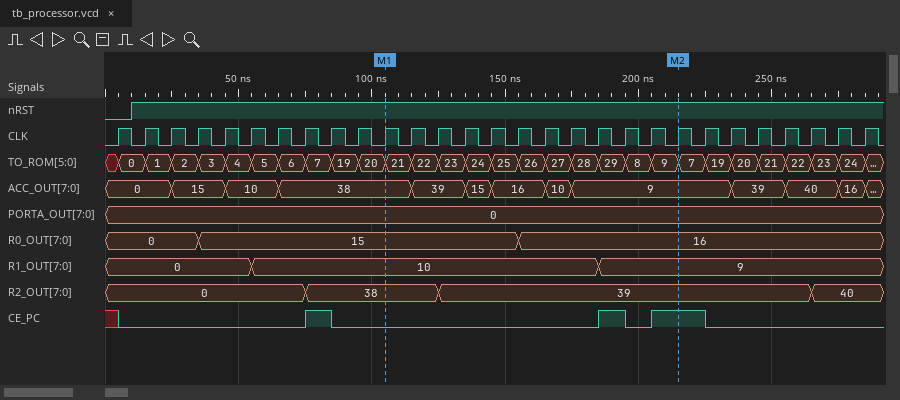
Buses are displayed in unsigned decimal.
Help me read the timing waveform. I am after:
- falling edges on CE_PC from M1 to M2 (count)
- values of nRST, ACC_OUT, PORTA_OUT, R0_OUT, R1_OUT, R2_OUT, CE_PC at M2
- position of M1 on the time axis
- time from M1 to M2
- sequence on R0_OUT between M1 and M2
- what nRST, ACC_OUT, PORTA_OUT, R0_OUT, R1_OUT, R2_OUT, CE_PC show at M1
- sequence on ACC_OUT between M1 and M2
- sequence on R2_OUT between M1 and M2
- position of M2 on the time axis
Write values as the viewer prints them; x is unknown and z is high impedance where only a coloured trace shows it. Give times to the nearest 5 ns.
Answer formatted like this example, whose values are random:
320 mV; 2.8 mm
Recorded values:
1; nRST=1, ACC_OUT=9, PORTA_OUT=0, R0_OUT=16, R1_OUT=9, R2_OUT=39, CE_PC=1; 105 ns; 110 ns; 15, 16; nRST=1, ACC_OUT=38, PORTA_OUT=0, R0_OUT=15, R1_OUT=10, R2_OUT=38, CE_PC=0; 38, 39, 15, 16, 10, 9; 38, 39; 215 ns
